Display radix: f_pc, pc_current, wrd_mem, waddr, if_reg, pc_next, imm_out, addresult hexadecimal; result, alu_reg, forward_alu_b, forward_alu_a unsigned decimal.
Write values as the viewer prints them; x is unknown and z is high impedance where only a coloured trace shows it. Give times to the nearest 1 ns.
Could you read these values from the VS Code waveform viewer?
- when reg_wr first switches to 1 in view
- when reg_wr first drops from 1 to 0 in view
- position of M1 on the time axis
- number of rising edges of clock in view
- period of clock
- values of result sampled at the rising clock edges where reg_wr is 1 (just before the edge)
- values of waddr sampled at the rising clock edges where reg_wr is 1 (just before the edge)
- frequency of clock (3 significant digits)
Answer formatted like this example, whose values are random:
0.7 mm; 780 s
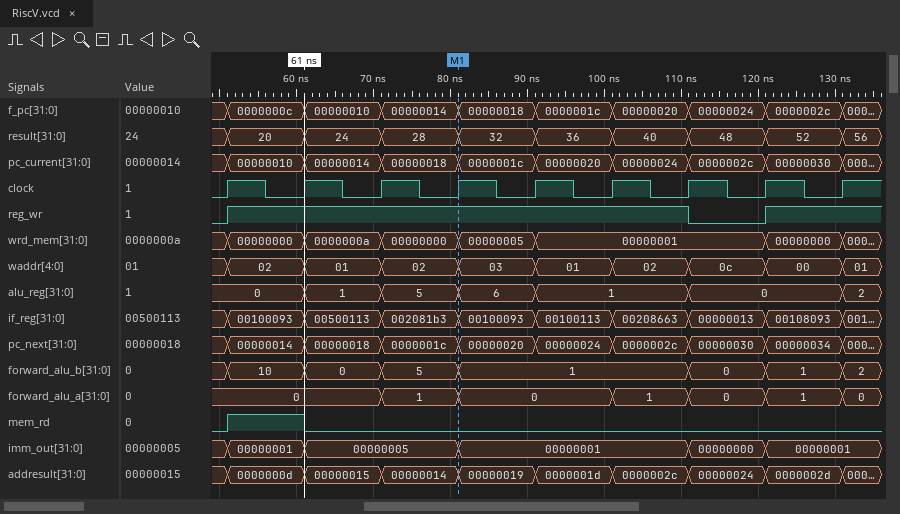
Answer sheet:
51 ns; 111 ns; 81 ns; 9; 10 ns; 20, 24, 28, 32, 36, 40, 52; 02, 01, 02, 03, 01, 02, 00; 100 MHz
